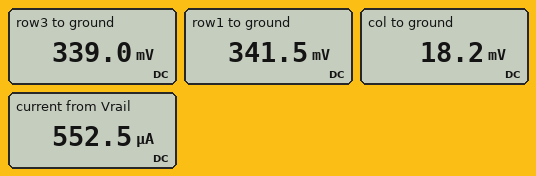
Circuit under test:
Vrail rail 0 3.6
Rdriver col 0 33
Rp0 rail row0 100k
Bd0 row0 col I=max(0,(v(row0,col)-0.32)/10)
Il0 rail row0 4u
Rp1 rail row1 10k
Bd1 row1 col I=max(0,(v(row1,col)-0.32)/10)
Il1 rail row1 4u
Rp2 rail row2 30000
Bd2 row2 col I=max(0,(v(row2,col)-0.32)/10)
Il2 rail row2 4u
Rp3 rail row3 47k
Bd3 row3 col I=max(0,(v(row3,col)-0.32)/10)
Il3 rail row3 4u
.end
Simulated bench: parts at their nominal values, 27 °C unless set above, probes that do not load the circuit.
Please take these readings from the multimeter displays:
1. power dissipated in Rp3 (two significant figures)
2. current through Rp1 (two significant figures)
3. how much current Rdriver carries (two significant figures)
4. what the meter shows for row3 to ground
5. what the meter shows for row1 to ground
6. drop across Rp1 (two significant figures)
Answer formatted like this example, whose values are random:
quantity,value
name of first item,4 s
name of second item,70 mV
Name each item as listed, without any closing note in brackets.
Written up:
quantity,value
power dissipated in Rp3,230 µW
current through Rp1,330 µA
how much current Rdriver carries,550 µA
what the meter shows for row3 to ground,339.0 mV
what the meter shows for row1 to ground,341.5 mV
drop across Rp1,3.3 V
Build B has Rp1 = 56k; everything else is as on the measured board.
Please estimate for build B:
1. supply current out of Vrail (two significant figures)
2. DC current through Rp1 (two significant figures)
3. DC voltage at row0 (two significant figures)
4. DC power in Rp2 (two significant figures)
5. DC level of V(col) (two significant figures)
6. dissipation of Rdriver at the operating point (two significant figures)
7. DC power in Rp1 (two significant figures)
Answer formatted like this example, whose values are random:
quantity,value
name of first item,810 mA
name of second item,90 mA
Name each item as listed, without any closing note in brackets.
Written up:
quantity,value
supply current out of Vrail,290 µA
DC current through Rp1,58 µA
DC voltage at row0,330 mV
DC power in Rp2,360 µW
DC level of V(col),9.4 mV
dissipation of Rdriver at the operating point,2.7 µW
DC power in Rp1,190 µW
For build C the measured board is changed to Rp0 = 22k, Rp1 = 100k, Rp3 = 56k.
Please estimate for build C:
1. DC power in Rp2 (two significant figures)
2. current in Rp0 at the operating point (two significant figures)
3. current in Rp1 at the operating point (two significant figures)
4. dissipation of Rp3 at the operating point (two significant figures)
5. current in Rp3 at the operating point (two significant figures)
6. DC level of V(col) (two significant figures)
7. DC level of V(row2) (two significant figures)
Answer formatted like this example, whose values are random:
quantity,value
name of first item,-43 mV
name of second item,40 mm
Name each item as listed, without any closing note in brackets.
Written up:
quantity,value
DC power in Rp2,360 µW
current in Rp0 at the operating point,150 µA
current in Rp1 at the operating point,33 µA
dissipation of Rp3 at the operating point,190 µW
current in Rp3 at the operating point,58 µA
DC level of V(col),12 mV
DC level of V(row2),330 mV
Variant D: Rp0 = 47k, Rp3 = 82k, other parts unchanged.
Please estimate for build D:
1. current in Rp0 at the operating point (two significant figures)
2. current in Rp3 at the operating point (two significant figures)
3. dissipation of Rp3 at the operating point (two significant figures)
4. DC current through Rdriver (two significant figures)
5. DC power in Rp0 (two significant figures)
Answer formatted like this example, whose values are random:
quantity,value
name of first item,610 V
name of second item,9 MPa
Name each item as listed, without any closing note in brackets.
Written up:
quantity,value
current in Rp0 at the operating point,69 µA
current in Rp3 at the operating point,40 µA
dissipation of Rp3 at the operating point,130 µW
DC current through Rdriver,560 µA
DC power in Rp0,230 µW
